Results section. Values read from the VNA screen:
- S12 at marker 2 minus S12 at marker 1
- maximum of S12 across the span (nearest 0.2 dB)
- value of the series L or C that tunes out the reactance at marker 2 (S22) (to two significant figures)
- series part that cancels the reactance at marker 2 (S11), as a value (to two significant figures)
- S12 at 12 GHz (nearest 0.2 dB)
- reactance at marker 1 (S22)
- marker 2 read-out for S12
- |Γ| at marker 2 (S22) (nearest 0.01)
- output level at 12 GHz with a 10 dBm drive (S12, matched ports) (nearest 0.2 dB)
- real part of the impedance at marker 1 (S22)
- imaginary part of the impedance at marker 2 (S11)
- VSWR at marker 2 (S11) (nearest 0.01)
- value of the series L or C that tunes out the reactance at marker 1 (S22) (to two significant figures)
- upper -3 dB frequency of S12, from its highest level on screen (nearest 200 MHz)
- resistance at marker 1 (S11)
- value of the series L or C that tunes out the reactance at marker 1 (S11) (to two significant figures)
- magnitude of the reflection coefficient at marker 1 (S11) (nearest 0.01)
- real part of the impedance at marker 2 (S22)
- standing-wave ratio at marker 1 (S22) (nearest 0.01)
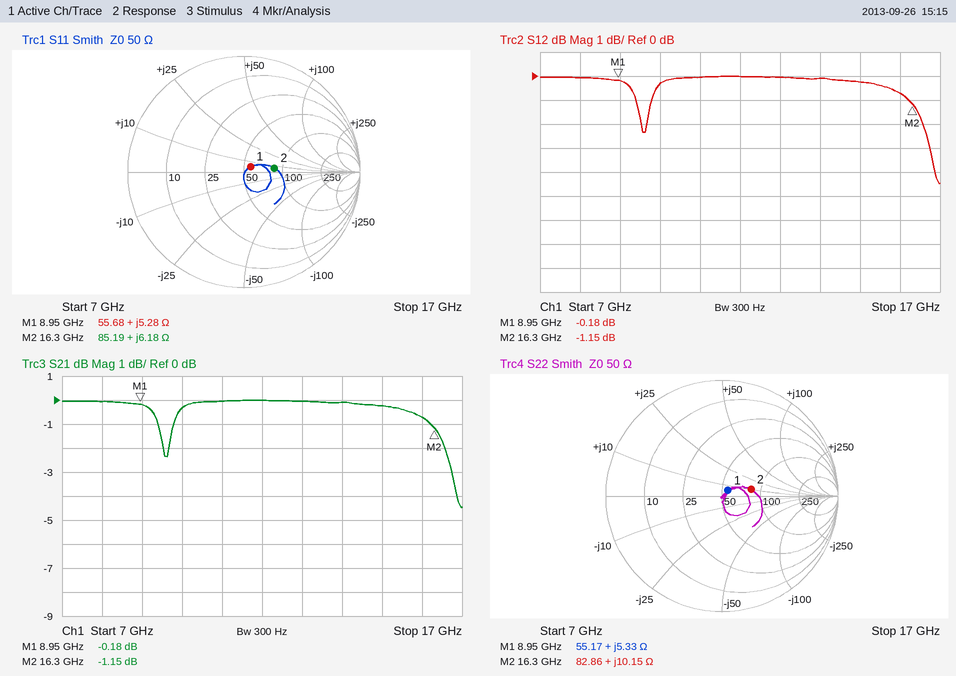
-0.97 dB
0.0 dB
960 fF
1.6 pF
0.0 dB
+5.33 Ω
-1.15 dB
0.26
10.0 dBm
55.17 Ω
+6.18 Ω
1.72
3.3 pF
16.8 GHz
55.68 Ω
3.4 pF
0.07
82.86 Ω
1.15
